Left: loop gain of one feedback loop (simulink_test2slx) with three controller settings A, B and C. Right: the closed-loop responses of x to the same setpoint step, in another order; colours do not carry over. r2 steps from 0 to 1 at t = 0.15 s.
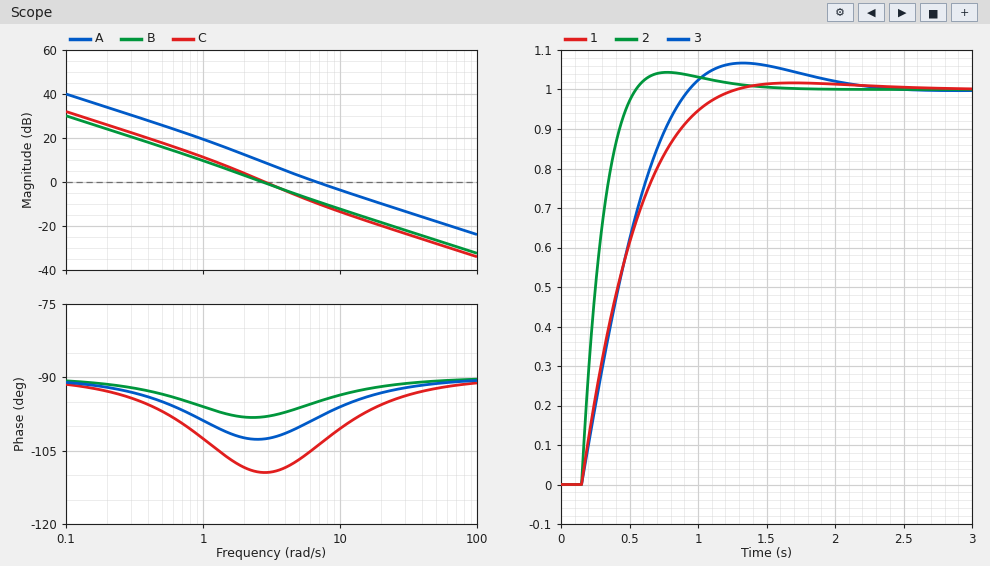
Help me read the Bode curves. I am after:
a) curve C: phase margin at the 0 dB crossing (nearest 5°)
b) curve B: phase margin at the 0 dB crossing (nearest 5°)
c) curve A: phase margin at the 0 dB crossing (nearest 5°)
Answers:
70°
80°
80°
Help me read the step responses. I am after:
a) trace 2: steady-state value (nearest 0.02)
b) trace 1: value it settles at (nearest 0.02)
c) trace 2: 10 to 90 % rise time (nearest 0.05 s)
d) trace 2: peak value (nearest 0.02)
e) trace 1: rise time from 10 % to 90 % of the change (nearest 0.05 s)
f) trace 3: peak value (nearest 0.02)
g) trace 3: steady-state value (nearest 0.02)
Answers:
1.00
1.00
0.25 s
1.04
0.70 s
1.06
1.00
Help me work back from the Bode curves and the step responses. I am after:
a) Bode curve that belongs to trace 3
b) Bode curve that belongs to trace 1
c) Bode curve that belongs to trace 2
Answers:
C
B
A
